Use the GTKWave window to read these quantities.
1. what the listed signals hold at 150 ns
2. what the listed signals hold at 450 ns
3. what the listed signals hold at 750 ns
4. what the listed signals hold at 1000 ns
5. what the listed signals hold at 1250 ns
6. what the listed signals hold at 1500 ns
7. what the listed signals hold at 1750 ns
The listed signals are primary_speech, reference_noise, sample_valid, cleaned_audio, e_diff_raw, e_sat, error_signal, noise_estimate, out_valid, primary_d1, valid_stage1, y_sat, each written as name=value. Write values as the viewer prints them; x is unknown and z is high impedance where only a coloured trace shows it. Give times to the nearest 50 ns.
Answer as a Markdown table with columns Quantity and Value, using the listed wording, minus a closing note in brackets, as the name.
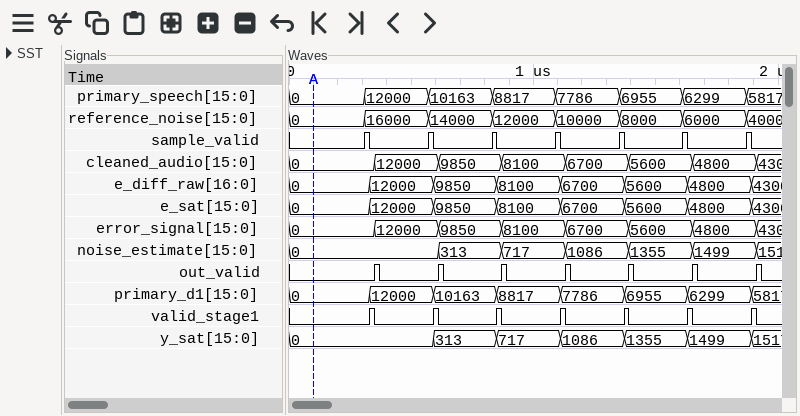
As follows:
| Quantity | Value |
|---|---|
| what the listed signals hold at 150 ns | primary_speech=0, reference_noise=0, sample_valid=0, cleaned_audio=0, e_diff_raw=0, e_sat=0, error_signal=0, noise_estimate=0, out_valid=0, primary_d1=0, valid_stage1=0, y_sat=0 |
| what the listed signals hold at 450 ns | primary_speech=12000, reference_noise=16000, sample_valid=0, cleaned_audio=12000, e_diff_raw=12000, e_sat=12000, error_signal=12000, noise_estimate=0, out_valid=0, primary_d1=12000, valid_stage1=0, y_sat=0 |
| what the listed signals hold at 750 ns | primary_speech=10163, reference_noise=14000, sample_valid=0, cleaned_audio=9850, e_diff_raw=9850, e_sat=9850, error_signal=9850, noise_estimate=313, out_valid=0, primary_d1=10163, valid_stage1=0, y_sat=313 |
| what the listed signals hold at 1000 ns | primary_speech=8817, reference_noise=12000, sample_valid=0, cleaned_audio=8100, e_diff_raw=8100, e_sat=8100, error_signal=8100, noise_estimate=717, out_valid=0, primary_d1=8817, valid_stage1=0, y_sat=717 |
| what the listed signals hold at 1250 ns | primary_speech=7786, reference_noise=10000, sample_valid=0, cleaned_audio=6700, e_diff_raw=6700, e_sat=6700, error_signal=6700, noise_estimate=1086, out_valid=0, primary_d1=7786, valid_stage1=0, y_sat=1086 |
| what the listed signals hold at 1500 ns | primary_speech=6955, reference_noise=8000, sample_valid=0, cleaned_audio=5600, e_diff_raw=5600, e_sat=5600, error_signal=5600, noise_estimate=1355, out_valid=0, primary_d1=6955, valid_stage1=0, y_sat=1355 |
| what the listed signals hold at 1750 ns | primary_speech=6299, reference_noise=6000, sample_valid=0, cleaned_audio=4800, e_diff_raw=4800, e_sat=4800, error_signal=4800, noise_estimate=1499, out_valid=0, primary_d1=6299, valid_stage1=0, y_sat=1499 |
